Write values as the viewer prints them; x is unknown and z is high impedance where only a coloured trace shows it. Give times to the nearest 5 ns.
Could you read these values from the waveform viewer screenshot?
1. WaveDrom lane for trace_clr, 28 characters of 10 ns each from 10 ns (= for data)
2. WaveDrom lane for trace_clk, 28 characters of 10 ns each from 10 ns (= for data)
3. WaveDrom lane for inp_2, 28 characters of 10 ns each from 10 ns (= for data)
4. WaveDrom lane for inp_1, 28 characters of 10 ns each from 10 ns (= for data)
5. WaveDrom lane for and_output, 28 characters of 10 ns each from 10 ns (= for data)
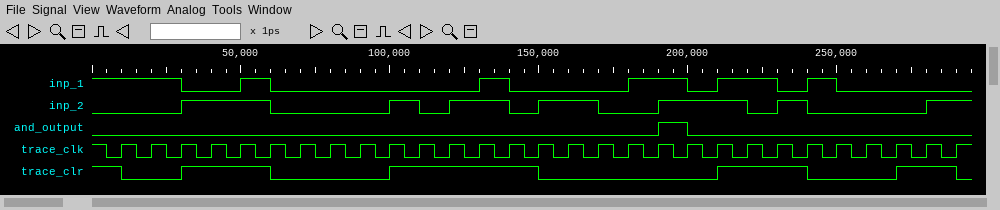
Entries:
{name: 'trace_clr', wave: '0.1..0...1....0.....1..0..1.'}
{name: 'trace_clk', wave: 'p...........................'}
{name: 'inp_2', wave: '0.1..0...101.01.0.1..010...1'}
{name: 'inp_1', wave: '1.0.10......10...1.01.010...'}
{name: 'and_output', wave: '0.................10........'}
